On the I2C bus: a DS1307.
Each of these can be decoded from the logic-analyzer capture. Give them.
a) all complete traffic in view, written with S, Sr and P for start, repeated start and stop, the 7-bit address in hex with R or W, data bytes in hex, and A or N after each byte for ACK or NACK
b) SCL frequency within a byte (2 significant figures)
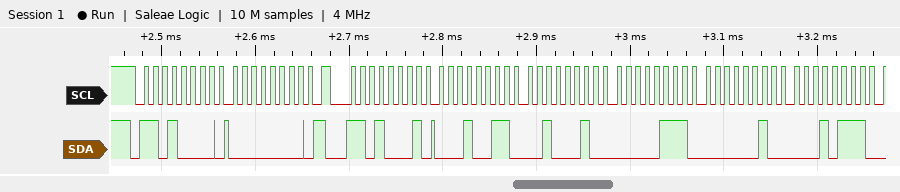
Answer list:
S 68W A 00 A Sr 68R A 13 A 22 A 07 A 02 A 17 A
100 kHz
